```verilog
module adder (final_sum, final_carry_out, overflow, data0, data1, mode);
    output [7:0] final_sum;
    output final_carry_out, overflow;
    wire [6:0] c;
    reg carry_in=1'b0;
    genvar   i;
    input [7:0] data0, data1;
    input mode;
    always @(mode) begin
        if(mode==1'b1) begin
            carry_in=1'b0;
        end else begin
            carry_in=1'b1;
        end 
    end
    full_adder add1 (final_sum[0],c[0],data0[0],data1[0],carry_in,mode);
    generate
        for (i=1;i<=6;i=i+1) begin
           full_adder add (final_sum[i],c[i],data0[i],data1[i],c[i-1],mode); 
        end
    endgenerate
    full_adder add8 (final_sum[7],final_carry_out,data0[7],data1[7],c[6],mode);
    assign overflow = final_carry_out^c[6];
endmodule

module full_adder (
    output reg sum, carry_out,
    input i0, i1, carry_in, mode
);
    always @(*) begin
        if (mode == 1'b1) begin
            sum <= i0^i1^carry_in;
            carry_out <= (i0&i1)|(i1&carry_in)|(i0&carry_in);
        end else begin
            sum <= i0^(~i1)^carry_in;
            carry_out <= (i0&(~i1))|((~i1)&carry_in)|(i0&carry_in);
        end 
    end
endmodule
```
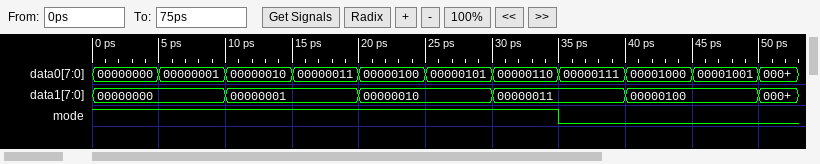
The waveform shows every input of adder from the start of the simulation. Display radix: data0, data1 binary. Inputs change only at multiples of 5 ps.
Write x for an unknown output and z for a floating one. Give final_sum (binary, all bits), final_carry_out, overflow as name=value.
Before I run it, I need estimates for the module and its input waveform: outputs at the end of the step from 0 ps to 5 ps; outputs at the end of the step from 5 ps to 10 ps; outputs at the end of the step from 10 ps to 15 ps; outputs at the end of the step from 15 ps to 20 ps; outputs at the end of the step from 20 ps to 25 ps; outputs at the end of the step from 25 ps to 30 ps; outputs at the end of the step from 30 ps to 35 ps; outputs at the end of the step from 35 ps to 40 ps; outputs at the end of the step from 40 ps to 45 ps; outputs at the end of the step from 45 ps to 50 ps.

final_sum=00000000, final_carry_out=0, overflow=0
final_sum=00000001, final_carry_out=0, overflow=0
final_sum=00000011, final_carry_out=0, overflow=0
final_sum=00000100, final_carry_out=0, overflow=0
final_sum=00000110, final_carry_out=0, overflow=0
final_sum=00000111, final_carry_out=0, overflow=0
final_sum=00001001, final_carry_out=0, overflow=0
final_sum=00000100, final_carry_out=1, overflow=0
final_sum=00000100, final_carry_out=1, overflow=0
final_sum=00000101, final_carry_out=1, overflow=0
